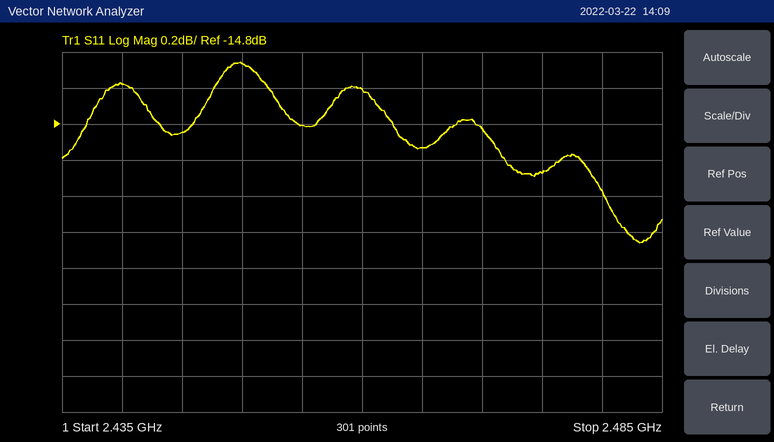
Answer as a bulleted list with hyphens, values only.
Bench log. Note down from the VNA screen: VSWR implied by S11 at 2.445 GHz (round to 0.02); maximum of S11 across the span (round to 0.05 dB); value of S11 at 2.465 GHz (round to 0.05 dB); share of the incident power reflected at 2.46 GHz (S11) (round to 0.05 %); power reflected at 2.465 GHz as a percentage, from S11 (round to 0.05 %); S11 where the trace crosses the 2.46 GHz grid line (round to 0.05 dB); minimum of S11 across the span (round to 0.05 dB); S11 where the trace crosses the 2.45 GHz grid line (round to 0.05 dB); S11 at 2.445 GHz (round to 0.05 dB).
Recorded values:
- 1.44
- -14.45 dB
- -14.95 dB
- 3.45 %
- 3.20 %
- -14.60 dB
- -15.45 dB
- -14.45 dB
- -14.85 dB
